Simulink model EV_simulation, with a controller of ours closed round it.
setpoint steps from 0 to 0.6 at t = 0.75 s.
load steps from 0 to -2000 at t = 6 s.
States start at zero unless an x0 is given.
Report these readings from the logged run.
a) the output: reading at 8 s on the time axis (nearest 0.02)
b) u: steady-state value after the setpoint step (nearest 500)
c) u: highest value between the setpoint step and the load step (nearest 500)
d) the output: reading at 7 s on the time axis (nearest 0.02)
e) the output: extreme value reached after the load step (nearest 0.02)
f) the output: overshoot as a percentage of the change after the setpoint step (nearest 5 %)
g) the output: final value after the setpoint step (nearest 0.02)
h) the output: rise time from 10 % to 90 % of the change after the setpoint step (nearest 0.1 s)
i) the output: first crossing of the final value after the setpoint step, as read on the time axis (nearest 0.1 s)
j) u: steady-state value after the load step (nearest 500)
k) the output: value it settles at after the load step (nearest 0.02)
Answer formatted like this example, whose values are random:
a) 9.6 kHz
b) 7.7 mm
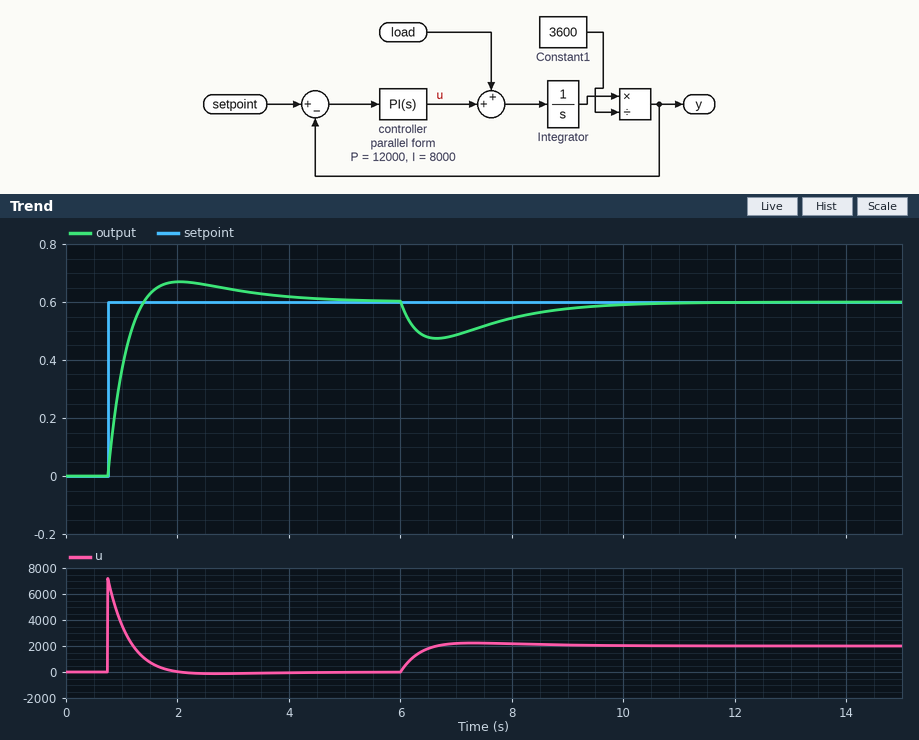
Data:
a) 0.54
b) 0
c) 7000
d) 0.48
e) 0.48
f) 10 %
g) 0.60
h) 0.5 s
i) 1.4 s
j) 2000
k) 0.60
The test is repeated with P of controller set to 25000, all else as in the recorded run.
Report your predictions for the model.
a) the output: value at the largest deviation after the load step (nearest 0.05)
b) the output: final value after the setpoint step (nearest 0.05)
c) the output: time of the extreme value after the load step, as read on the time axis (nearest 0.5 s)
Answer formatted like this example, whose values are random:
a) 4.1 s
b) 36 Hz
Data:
a) 0.55
b) 0.60
c) 6.5 s
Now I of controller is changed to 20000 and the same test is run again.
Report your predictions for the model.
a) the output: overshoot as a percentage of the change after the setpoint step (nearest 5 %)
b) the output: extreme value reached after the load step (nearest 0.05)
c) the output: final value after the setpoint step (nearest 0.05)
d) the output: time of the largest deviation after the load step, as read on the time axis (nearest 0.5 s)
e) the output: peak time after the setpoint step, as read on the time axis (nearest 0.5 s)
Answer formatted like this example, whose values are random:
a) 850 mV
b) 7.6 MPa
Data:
a) 20 %
b) 0.50
c) 0.60
d) 6.5 s
e) 1.5 s
